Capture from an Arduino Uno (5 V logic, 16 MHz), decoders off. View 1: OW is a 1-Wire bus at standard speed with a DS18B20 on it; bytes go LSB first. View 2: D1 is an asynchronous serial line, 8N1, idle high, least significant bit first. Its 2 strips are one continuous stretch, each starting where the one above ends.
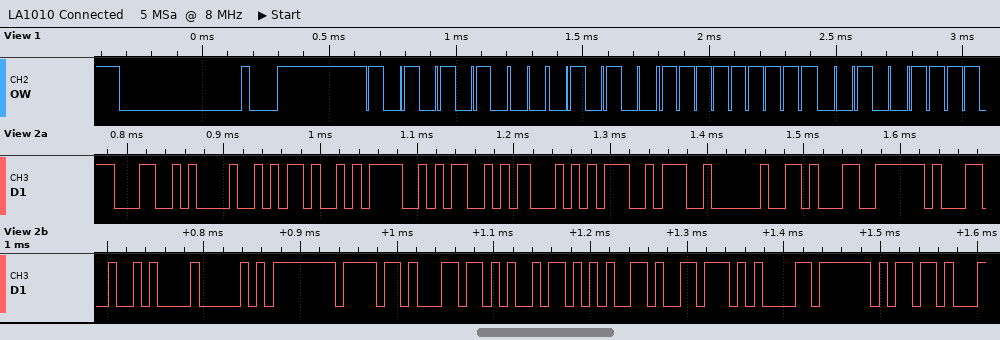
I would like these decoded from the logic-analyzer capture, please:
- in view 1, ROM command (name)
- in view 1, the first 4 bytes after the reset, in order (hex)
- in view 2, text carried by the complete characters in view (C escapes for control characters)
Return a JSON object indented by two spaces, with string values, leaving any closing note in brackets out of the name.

{
  "in view 1, ROM command": "Match ROM",
  "in view 1, the first 4 bytes after the reset, in order": "55 28 FF C9",
  "in view 2, text carried by the complete characters in view": "\"LHKOST: 11\\nPolievam\""
}
